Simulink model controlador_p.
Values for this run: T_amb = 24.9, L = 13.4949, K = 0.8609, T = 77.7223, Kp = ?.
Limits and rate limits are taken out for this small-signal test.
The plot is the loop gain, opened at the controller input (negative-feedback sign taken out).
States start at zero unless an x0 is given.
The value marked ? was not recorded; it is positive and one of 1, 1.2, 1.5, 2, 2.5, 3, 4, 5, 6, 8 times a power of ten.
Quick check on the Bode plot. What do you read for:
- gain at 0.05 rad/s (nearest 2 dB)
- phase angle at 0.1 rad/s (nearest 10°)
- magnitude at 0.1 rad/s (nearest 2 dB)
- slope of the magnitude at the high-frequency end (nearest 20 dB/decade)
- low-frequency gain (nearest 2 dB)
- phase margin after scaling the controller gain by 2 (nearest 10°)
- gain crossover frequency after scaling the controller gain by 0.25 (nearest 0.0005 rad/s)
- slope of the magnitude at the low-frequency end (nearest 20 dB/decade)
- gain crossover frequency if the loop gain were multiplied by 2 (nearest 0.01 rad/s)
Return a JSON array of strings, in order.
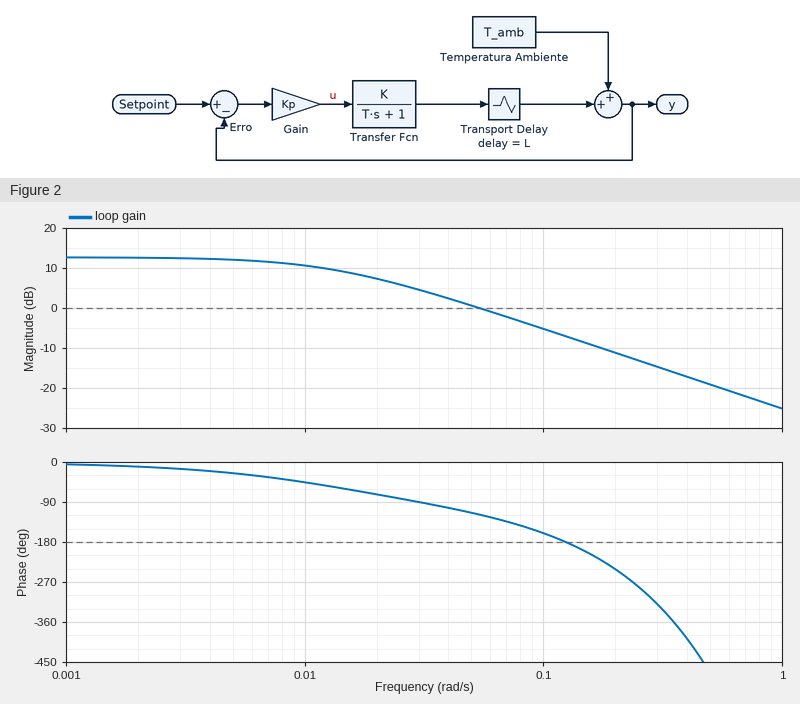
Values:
["0 dB", "-160°", "-6 dB", "-20 dB/decade", "12 dB", "10°", "0.0050 rad/s", "0 dB/decade", "0.11 rad/s"]
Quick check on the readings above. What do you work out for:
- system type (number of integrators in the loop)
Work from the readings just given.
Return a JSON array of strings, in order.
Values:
["0"]
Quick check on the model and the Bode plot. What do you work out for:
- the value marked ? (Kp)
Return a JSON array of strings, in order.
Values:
["5"]
